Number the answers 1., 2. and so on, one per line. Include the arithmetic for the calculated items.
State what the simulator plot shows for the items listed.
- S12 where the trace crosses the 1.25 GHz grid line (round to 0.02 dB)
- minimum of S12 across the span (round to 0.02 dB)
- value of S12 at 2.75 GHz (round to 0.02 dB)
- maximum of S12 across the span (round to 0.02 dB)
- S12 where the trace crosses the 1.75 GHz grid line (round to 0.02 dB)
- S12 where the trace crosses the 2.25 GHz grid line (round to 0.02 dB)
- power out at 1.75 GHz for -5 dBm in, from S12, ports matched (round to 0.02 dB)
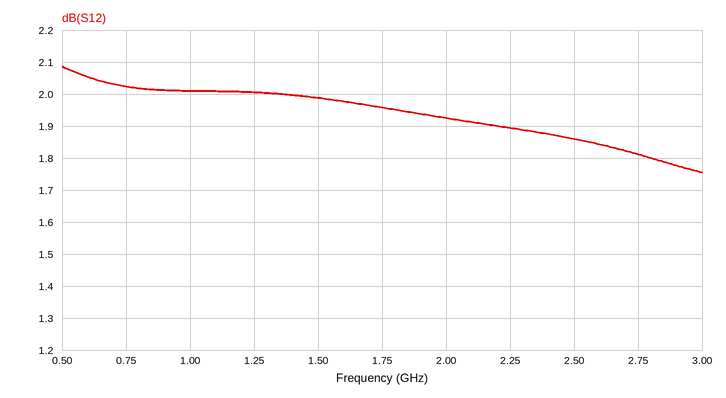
1. 2.00 dB
2. 1.76 dB
3. 1.82 dB
4. 2.08 dB
5. 1.96 dB
6. 1.90 dB
7. -5 dBm + (1.96 dB) = -3.04 dBm
